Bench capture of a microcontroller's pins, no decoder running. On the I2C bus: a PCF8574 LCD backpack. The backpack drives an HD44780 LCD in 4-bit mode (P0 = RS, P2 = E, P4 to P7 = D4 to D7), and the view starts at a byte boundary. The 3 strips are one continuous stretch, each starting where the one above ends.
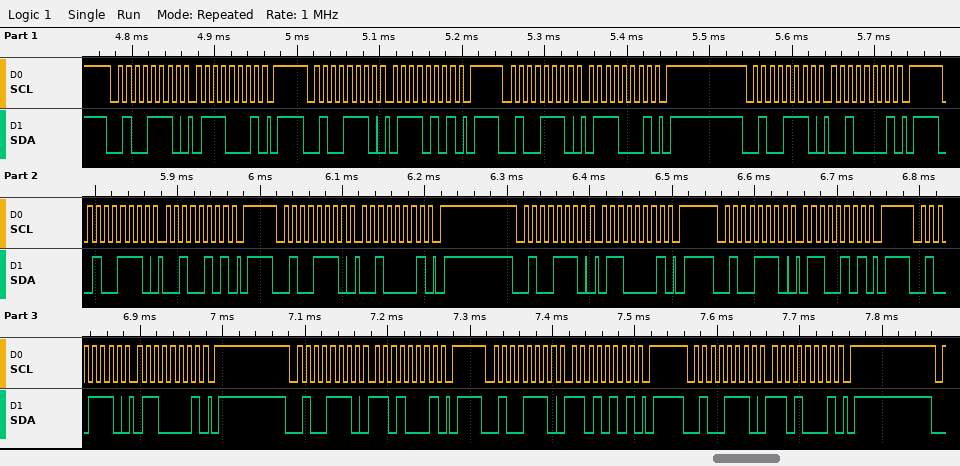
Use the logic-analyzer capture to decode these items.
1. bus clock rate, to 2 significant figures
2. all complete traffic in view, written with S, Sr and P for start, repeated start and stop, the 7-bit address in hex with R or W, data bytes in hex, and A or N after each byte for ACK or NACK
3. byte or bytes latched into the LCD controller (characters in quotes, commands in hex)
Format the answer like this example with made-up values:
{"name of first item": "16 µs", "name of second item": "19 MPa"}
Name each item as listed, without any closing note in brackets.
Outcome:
{"bus clock rate, to 2 significant figures": "100 kHz", "all complete traffic in view, written with S, Sr and P for start, repeated start and stop, the 7-bit address in hex with R or W, data bytes in hex, and A or N after each byte for ACK or NACK": "S 27W A 71 A P S 27W A 75 A P S 27W A 71 A P S 27W A 21 A P S 27W A 25 A P S 27W A 21 A P S 27W A 61 A P S 27W A 65 A P S 27W A 61 A P S 27W A D1 A P S 27W A D5 A P S 27W A D1 A P", "byte or bytes latched into the LCD controller": "'r' 'm'"}
